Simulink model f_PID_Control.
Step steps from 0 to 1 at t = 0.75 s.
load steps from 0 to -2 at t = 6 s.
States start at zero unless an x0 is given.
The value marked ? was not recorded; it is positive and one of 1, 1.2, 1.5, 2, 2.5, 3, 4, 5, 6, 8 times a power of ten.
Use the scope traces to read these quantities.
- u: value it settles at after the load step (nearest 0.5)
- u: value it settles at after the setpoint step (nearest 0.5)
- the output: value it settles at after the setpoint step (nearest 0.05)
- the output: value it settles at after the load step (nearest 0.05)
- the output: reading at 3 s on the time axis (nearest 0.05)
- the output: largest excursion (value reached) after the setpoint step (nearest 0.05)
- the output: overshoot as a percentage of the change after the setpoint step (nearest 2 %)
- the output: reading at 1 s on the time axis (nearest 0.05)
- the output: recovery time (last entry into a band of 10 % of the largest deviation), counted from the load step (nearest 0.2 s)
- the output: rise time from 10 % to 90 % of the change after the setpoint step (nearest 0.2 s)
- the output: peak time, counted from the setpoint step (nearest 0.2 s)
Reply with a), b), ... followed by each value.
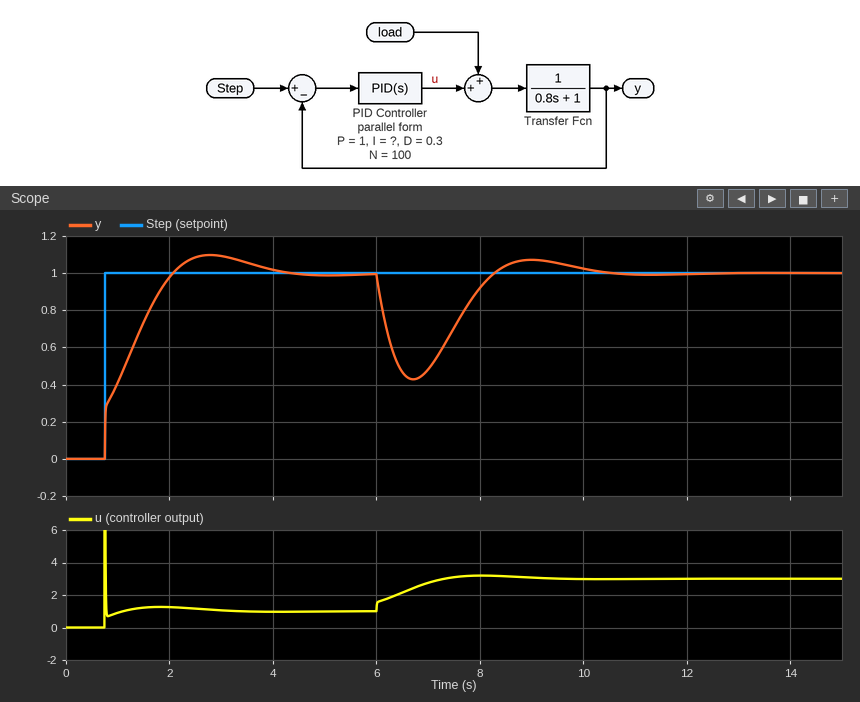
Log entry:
a) 3.0
b) 1.0
c) 1.00
d) 1.00
e) 1.10
f) 1.10
g) 10 %
h) 0.40
i) 3.4 s
j) 1.0 s
k) 2.0 s
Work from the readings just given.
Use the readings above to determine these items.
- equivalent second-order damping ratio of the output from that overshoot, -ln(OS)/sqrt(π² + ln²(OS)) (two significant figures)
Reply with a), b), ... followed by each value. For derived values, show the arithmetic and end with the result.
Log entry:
a) ln(0.1) = -2.303; 2.303 / sqrt(9.870 + 5.302) = 0.59
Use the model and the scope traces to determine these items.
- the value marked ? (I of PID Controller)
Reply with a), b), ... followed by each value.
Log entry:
a) 3
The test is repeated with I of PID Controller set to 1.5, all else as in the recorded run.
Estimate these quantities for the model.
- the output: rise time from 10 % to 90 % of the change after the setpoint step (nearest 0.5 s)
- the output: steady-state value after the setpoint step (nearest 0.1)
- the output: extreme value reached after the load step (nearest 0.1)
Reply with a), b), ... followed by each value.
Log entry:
a) 2.0 s
b) 1.0
c) 0.3
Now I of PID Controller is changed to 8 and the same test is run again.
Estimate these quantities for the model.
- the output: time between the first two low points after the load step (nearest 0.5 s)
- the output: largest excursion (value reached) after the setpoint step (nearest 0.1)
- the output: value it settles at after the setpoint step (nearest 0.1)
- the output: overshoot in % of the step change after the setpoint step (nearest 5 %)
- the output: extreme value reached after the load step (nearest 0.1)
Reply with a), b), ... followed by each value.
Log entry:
a) 2.5 s
b) 1.2
c) 1.0
d) 25 %
e) 0.6
